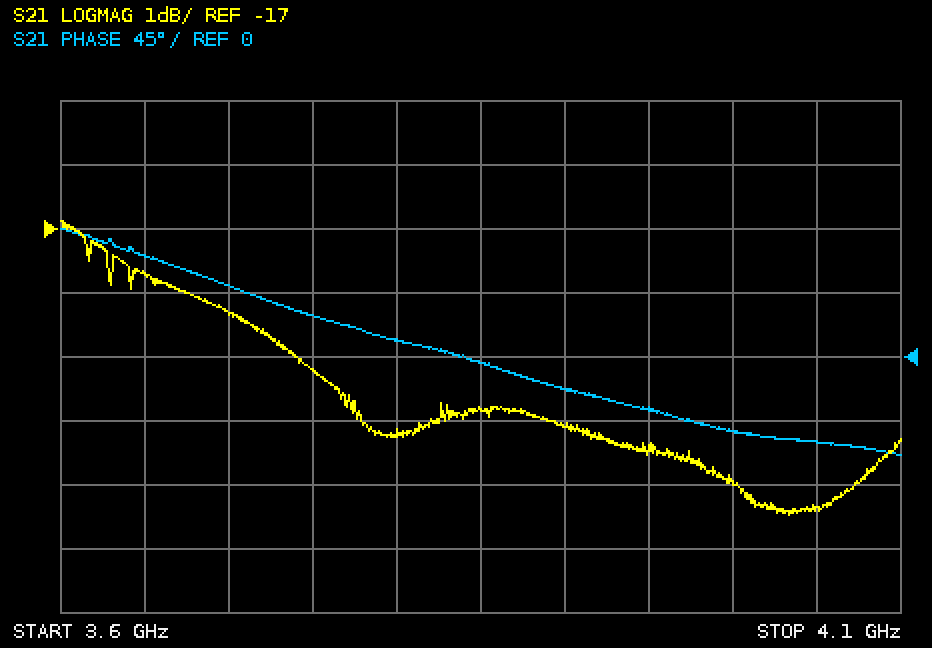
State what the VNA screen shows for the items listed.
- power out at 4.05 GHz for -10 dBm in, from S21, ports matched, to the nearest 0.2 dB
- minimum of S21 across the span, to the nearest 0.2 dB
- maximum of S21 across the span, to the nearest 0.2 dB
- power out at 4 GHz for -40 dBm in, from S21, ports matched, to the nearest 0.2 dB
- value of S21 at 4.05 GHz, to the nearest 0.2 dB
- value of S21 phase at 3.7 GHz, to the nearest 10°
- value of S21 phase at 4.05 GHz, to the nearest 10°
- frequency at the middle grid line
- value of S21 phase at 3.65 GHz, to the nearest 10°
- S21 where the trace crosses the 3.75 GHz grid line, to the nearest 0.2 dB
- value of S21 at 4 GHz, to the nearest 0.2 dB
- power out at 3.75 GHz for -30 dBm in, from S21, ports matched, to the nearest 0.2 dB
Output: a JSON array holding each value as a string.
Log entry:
["-31.4 dBm", "-21.4 dB", "-16.8 dB", "-61.0 dBm", "-21.4 dB", "50°", "-60°", "3.85 GHz", "70°", "-19.2 dB", "-21.0 dB", "-49.2 dBm"]
